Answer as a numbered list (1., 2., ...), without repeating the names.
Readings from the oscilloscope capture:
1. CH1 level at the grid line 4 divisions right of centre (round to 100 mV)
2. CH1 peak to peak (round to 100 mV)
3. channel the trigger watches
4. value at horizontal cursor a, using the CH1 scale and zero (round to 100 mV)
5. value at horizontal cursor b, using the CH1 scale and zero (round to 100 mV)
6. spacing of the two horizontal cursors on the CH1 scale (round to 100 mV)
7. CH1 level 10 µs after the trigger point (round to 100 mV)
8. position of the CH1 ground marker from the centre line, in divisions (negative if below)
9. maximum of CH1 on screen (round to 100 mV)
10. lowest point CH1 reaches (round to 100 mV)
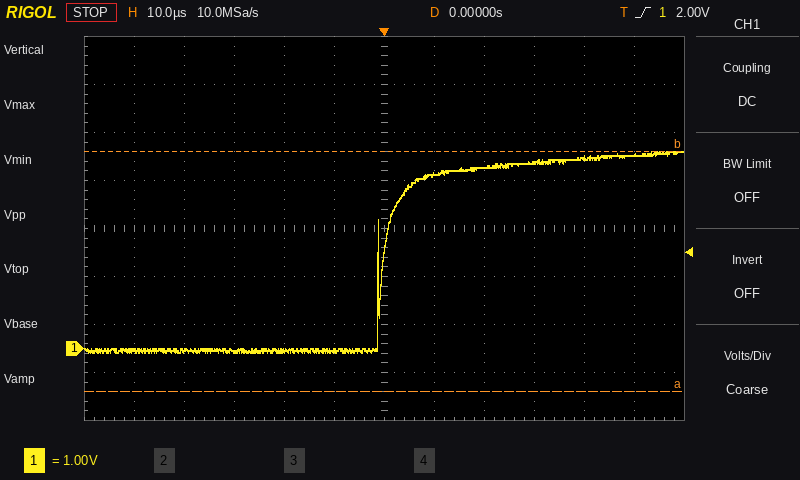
1. 4.0 V
2. 4.2 V
3. CH1
4. -900 mV
5. 4.1 V
6. 5.0 V
7. 3.6 V
8. -2.5 div
9. 4.1 V
10. -100 mV
